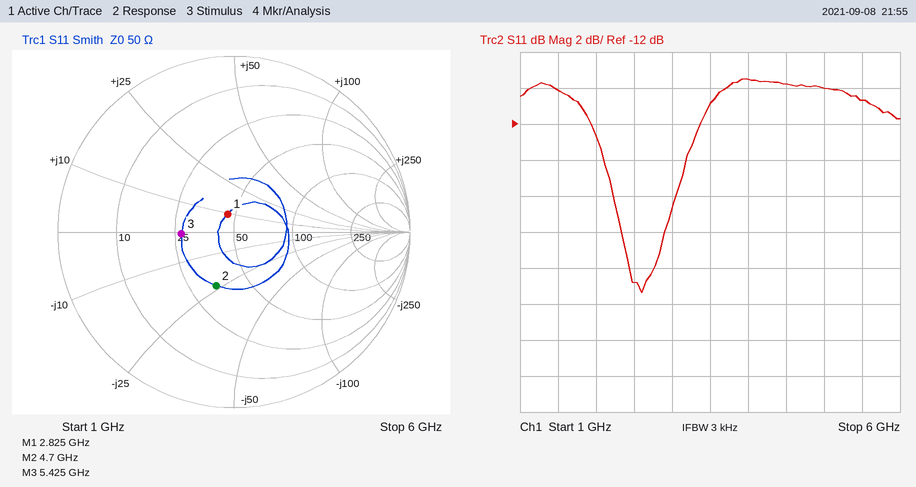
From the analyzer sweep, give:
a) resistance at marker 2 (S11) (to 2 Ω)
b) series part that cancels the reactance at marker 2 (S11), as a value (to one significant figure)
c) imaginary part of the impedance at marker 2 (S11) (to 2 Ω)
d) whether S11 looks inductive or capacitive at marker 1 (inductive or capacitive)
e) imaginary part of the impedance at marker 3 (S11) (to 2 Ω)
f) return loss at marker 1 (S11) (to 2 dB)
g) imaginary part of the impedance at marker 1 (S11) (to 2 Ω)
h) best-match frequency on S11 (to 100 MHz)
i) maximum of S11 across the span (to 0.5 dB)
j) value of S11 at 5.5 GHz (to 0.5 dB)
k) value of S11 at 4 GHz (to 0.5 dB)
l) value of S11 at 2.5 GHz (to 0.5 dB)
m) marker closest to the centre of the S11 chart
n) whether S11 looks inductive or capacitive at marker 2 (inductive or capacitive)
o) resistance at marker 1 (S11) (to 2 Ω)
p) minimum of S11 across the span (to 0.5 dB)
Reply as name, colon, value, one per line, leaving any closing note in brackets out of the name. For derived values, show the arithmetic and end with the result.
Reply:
resistance at marker 2 (S11): 34 Ω
series part that cancels the reactance at marker 2 (S11), as a value: L = 24 Ω/(2π × 4.7 GHz) ≈ 813 pH, so 800 pH to one significant figure
imaginary part of the impedance at marker 2 (S11): -24 Ω
whether S11 looks inductive or capacitive at marker 1: inductive
imaginary part of the impedance at marker 3 (S11): 0 Ω
return loss at marker 1 (S11): 20 dB
imaginary part of the impedance at marker 1 (S11): +10 Ω
best-match frequency on S11: 2.6 GHz
maximum of S11 across the span: -9.5 dB
value of S11 at 5.5 GHz: -10.5 dB
value of S11 at 4 GHz: -9.5 dB
value of S11 at 2.5 GHz: -21.0 dB
marker closest to the centre of the S11 chart: marker 1
whether S11 looks inductive or capacitive at marker 2: capacitive
resistance at marker 1 (S11): 46 Ω
minimum of S11 across the span: -21.5 dB
